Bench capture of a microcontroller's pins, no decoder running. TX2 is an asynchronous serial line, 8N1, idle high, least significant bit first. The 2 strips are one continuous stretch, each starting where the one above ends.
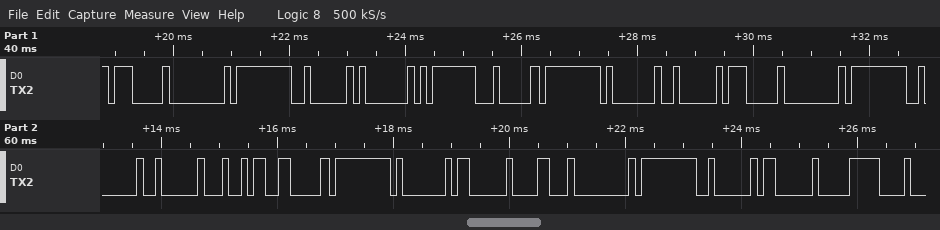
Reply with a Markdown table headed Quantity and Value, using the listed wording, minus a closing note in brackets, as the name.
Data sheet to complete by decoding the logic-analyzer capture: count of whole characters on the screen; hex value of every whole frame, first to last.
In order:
| Quantity | Value |
|---|---|
| count of whole characters on the screen | 26 |
| hex value of every whole frame, first to last | 07 00 FF 02 01 FD 04 FF 01 02 07 00 FF 02 02 A4 06 FF 01 03 18 00 FF 02 03 F0 |
